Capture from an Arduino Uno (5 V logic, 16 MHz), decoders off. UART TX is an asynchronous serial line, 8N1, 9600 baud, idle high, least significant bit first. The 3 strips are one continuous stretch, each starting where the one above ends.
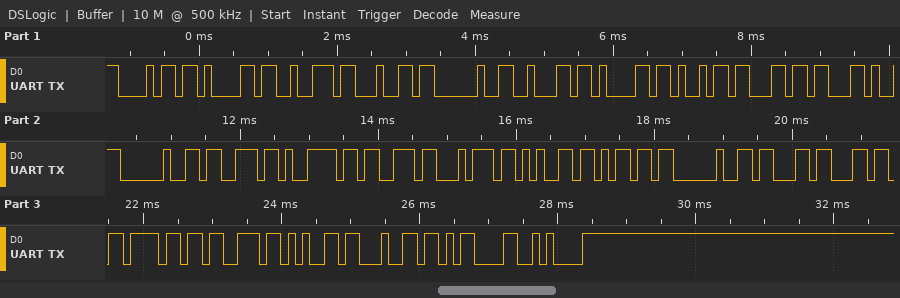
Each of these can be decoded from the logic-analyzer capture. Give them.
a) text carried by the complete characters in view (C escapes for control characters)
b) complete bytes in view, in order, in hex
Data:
"hard bail, system closed\r\n"
68 61 72 64 20 62 61 69 6C 2C 20 73 79 73 74 65 6D 20 63 6C 6F 73 65 64 0D 0A
